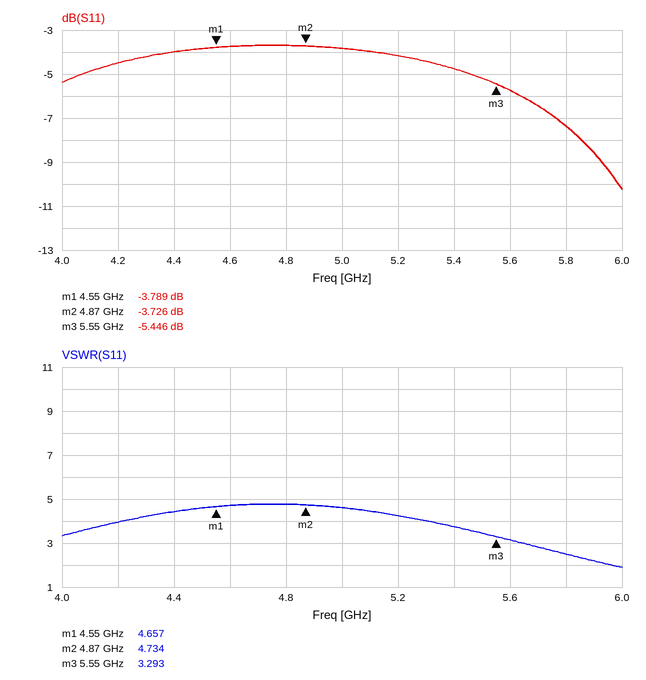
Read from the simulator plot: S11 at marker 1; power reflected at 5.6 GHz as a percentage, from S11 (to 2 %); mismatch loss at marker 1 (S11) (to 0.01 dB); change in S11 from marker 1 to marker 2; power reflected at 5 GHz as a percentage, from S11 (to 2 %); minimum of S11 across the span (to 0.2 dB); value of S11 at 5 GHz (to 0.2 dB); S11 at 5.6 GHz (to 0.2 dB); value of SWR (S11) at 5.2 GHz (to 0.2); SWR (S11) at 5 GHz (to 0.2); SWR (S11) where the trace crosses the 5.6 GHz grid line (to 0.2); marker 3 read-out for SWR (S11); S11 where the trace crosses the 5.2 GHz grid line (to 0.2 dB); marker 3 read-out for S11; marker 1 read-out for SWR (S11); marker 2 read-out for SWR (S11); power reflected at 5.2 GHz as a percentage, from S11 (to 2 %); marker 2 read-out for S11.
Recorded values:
-3.789 dB
26 %
2.35 dB
0.063 dB
42 %
-10.2 dB
-3.8 dB
-5.8 dB
4.2
4.6
3.2
3.293
-4.2 dB
-5.446 dB
4.657
4.734
38 %
-3.726 dB
